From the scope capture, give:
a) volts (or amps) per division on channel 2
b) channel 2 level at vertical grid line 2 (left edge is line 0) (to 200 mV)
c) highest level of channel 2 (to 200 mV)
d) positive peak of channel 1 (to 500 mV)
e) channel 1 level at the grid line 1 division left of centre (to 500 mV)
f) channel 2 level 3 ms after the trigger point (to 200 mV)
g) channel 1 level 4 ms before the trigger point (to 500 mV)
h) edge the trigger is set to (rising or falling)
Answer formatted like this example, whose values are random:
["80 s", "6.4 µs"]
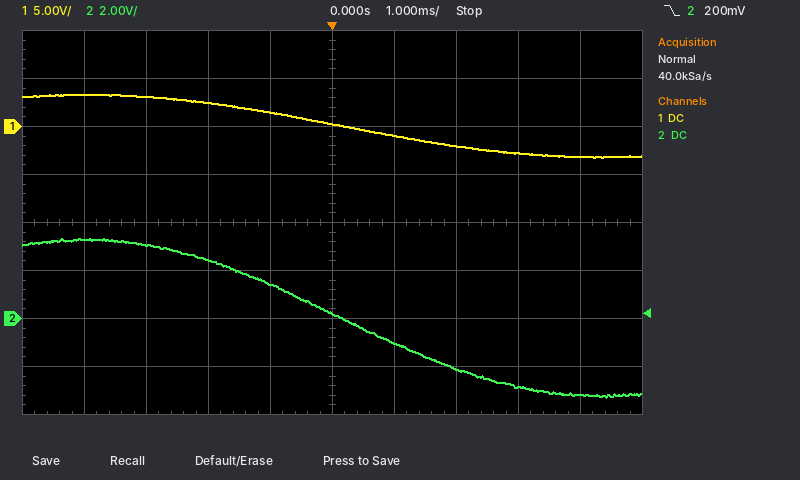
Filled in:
["2 V", "3.0 V", "3.4 V", "3.5 V", "1.5 V", "-2.8 V", "3.5 V", "falling"]
